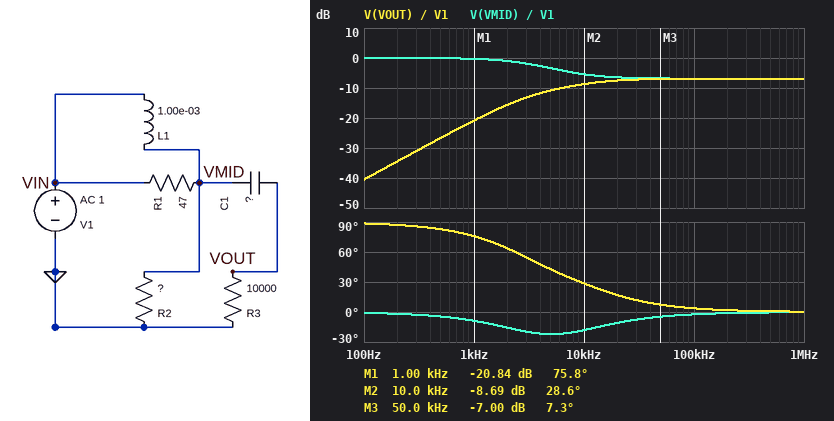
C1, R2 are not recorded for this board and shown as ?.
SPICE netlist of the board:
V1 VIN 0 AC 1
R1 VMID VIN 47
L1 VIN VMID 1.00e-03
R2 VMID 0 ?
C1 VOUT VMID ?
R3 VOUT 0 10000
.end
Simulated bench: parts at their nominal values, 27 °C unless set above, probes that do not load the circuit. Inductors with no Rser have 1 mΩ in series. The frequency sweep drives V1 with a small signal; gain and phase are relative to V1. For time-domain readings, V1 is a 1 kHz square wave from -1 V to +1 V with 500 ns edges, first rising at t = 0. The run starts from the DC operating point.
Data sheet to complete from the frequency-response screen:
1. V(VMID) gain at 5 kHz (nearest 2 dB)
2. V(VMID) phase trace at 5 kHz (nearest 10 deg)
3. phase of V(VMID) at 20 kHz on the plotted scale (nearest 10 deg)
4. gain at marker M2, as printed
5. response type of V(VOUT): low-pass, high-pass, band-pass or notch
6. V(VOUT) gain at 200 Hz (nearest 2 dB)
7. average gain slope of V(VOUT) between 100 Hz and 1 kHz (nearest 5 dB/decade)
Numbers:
-4 dB
-20 deg
-10 deg
-8.69 dB
high-pass
-34 dB
20 dB/decade
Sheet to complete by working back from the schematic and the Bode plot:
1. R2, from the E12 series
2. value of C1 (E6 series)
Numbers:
39 Ω
1.5 nF
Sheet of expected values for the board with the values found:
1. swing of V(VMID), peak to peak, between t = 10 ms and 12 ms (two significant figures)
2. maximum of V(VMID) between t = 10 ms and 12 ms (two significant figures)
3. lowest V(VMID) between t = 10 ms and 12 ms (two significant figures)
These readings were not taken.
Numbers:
2.0 V
1.0 V
-1.0 V
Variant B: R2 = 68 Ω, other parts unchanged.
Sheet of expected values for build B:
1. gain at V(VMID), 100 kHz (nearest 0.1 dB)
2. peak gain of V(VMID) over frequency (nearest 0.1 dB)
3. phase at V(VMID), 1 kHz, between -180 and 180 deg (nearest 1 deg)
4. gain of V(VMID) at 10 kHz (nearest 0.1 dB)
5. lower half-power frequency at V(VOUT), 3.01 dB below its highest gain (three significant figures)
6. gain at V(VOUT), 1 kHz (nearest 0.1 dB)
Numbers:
-4.6 dB
0 dB
-5 deg
-3.4 dB
7.58 kHz
-20.7 dB
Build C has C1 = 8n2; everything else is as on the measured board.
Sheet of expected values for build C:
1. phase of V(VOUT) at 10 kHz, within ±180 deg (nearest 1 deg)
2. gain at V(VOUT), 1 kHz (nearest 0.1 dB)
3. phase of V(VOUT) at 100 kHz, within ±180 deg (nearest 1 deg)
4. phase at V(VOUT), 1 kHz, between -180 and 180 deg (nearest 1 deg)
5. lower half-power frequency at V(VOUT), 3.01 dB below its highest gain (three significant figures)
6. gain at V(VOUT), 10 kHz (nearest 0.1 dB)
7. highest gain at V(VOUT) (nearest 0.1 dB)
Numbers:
-7 deg
-7.1 dB
-1 deg
54 deg
1.12 kHz
-5.6 dB
-3.4 dB
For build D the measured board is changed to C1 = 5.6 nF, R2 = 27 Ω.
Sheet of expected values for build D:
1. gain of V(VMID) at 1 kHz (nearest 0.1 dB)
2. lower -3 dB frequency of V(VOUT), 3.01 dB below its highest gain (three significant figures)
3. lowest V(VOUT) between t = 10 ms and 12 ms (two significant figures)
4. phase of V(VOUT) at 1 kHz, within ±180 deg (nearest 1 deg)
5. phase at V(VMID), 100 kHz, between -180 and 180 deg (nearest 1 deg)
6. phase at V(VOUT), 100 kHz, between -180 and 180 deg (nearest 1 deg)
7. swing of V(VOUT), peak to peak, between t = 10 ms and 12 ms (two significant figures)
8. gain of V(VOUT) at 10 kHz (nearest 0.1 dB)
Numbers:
-0.5 dB
1.26 kHz
-820 mV
58 deg
-3 deg
-1 deg
1.6 V
-7.5 dB
